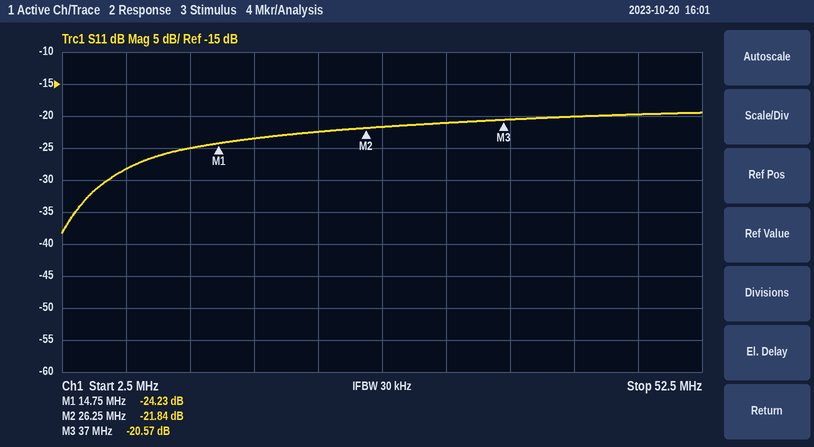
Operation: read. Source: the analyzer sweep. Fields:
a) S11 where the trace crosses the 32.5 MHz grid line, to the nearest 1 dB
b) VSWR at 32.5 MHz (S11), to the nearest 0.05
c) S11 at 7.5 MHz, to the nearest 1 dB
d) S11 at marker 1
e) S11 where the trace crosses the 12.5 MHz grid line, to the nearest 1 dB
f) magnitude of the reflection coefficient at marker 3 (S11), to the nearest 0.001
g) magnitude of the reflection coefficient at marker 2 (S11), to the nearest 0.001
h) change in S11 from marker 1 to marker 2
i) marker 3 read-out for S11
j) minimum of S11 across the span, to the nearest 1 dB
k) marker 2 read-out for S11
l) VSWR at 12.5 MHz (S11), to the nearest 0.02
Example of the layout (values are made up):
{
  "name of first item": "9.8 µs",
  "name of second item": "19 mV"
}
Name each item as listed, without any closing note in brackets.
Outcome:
{
  "S11 where the trace crosses the 32.5 MHz grid line, to the nearest 1 dB": "-21 dB",
  "VSWR at 32.5 MHz (S11), to the nearest 0.05": "1.20",
  "S11 at 7.5 MHz, to the nearest 1 dB": "-28 dB",
  "S11 at marker 1": "-24.23 dB",
  "S11 where the trace crosses the 12.5 MHz grid line, to the nearest 1 dB": "-25 dB",
  "magnitude of the reflection coefficient at marker 3 (S11), to the nearest 0.001": "0.094",
  "magnitude of the reflection coefficient at marker 2 (S11), to the nearest 0.001": "0.081",
  "change in S11 from marker 1 to marker 2": "2.39 dB",
  "marker 3 read-out for S11": "-20.57 dB",
  "minimum of S11 across the span, to the nearest 1 dB": "-38 dB",
  "marker 2 read-out for S11": "-21.84 dB",
  "VSWR at 12.5 MHz (S11), to the nearest 0.02": "1.12"
}
